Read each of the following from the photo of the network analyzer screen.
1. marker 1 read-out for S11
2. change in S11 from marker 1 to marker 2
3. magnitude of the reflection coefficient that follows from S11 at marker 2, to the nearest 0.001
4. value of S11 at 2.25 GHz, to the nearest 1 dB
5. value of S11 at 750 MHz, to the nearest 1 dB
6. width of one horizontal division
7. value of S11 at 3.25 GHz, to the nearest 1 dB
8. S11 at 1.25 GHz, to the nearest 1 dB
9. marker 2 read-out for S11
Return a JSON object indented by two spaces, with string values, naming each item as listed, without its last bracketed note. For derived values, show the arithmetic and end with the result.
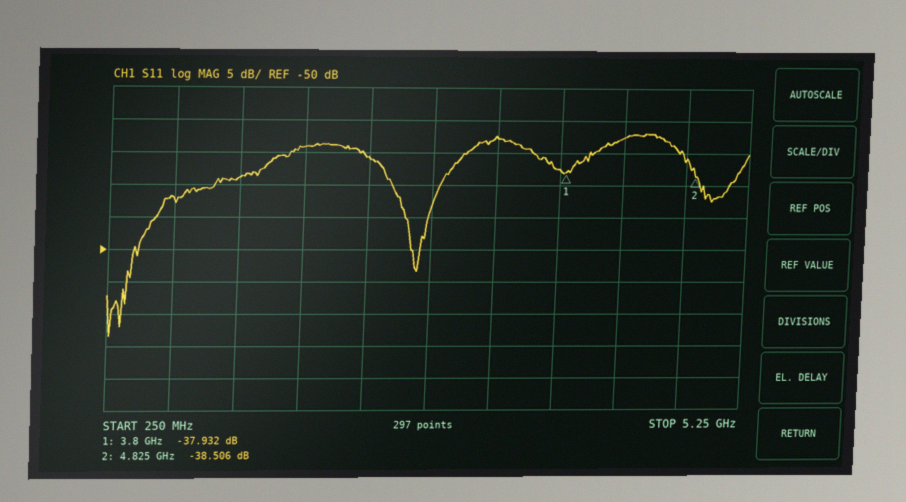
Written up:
{
  "marker 1 read-out for S11": "-37.932 dB",
  "change in S11 from marker 1 to marker 2": "-38.506 − (-37.932) = -0.574 dB",
  "magnitude of the reflection coefficient that follows from S11 at marker 2, to the nearest 0.001": "10^(-38.506/20) ≈ 0.012",
  "value of S11 at 2.25 GHz, to the nearest 1 dB": "-36 dB",
  "value of S11 at 750 MHz, to the nearest 1 dB": "-42 dB",
  "width of one horizontal division": "500 MHz",
  "value of S11 at 3.25 GHz, to the nearest 1 dB": "-33 dB",
  "S11 at 1.25 GHz, to the nearest 1 dB": "-39 dB",
  "marker 2 read-out for S11": "-38.506 dB"
}
